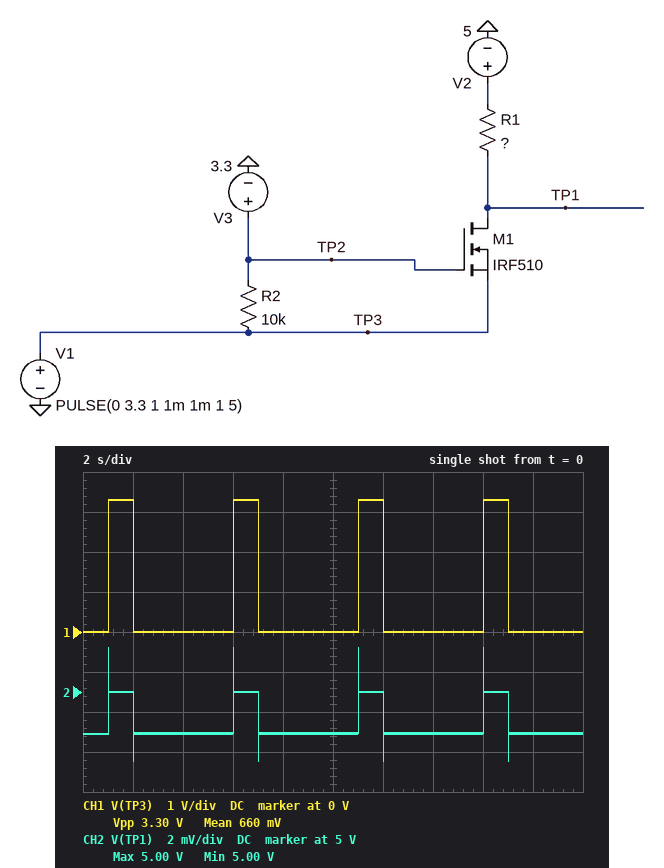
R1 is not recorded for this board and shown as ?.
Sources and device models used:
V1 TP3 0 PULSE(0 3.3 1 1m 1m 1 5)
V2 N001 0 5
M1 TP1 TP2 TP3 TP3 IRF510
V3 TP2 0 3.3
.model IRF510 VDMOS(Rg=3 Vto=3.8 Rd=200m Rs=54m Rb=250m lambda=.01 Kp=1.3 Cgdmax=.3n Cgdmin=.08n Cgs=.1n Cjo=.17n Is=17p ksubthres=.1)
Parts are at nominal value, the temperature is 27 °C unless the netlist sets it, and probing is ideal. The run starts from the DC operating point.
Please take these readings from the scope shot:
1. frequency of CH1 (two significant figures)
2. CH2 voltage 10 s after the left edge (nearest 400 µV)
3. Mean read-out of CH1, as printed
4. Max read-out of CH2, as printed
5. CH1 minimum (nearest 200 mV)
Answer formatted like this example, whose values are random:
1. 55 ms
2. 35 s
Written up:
1. 200 mHz
2. 4.9980 V
3. 660 mV
4. 5.00 V
5. 0 V
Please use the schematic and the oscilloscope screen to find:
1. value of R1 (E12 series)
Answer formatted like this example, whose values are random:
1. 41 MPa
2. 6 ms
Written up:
1. 6.8 kΩ
